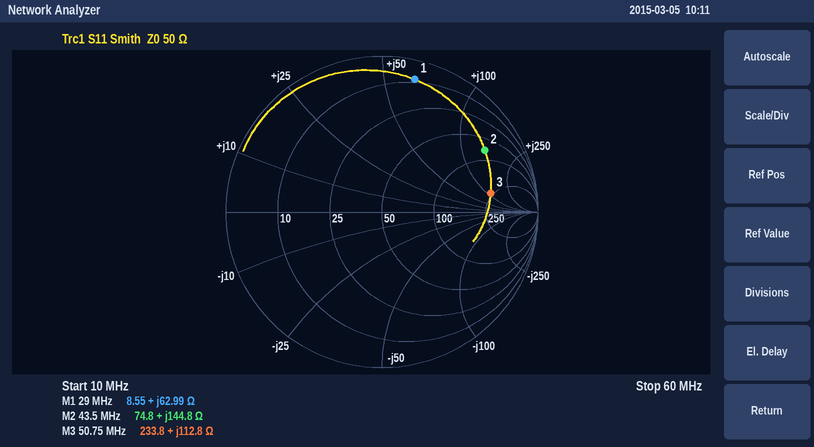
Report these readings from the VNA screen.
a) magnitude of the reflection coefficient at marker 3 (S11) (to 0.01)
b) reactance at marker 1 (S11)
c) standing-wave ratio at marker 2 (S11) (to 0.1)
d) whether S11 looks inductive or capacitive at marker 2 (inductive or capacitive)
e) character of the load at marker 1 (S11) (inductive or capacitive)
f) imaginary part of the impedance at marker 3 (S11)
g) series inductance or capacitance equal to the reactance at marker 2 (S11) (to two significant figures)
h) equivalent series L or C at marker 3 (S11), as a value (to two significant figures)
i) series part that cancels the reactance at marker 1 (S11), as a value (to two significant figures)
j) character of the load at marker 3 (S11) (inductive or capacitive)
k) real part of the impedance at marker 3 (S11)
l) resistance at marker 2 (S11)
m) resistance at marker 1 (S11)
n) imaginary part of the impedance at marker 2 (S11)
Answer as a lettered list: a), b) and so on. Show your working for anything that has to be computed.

a) 0.71
b) +62.99 Ω
c) 7.6
d) inductive
e) inductive
f) +112.8 Ω
g) L = 144.8 Ω/(2π × 43.5 MHz) ≈ 530 nH
h) L = 112.8 Ω/(2π × 50.75 MHz) ≈ 354 nH, so 350 nH to two significant figures
i) C = 1/(2π × 29 MHz × 62.99 Ω) ≈ 87 pF
j) inductive
k) 233.8 Ω
l) 74.8 Ω
m) 8.55 Ω
n) +144.8 Ω
